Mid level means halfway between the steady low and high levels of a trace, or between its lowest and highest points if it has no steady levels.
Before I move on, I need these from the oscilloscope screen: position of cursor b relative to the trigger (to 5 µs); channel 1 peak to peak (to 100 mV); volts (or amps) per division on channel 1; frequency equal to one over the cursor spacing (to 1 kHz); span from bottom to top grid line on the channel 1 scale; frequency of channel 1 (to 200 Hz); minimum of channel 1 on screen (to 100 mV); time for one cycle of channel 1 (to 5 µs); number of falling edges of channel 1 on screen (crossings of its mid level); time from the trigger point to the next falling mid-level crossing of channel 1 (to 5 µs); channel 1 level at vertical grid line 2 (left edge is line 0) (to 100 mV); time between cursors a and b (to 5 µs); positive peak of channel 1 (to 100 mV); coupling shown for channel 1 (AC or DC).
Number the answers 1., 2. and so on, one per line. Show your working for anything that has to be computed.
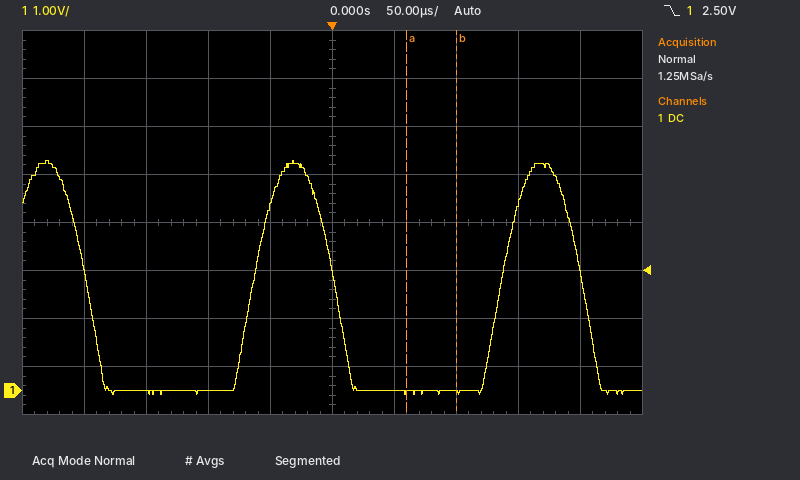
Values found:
1. +100 µs
2. 4.8 V − (-100 mV) = 4.9 V
3. 1 V
4. 1 / 40 µs ≈ 25 kHz
5. 8 V
6. 1 / 200 µs ≈ 5.0 kHz
7. -100 mV
8. 200 µs
9. 3
10. 200 µs
11. 0.0 V
12. 40 µs
13. 4.8 V
14. DC
